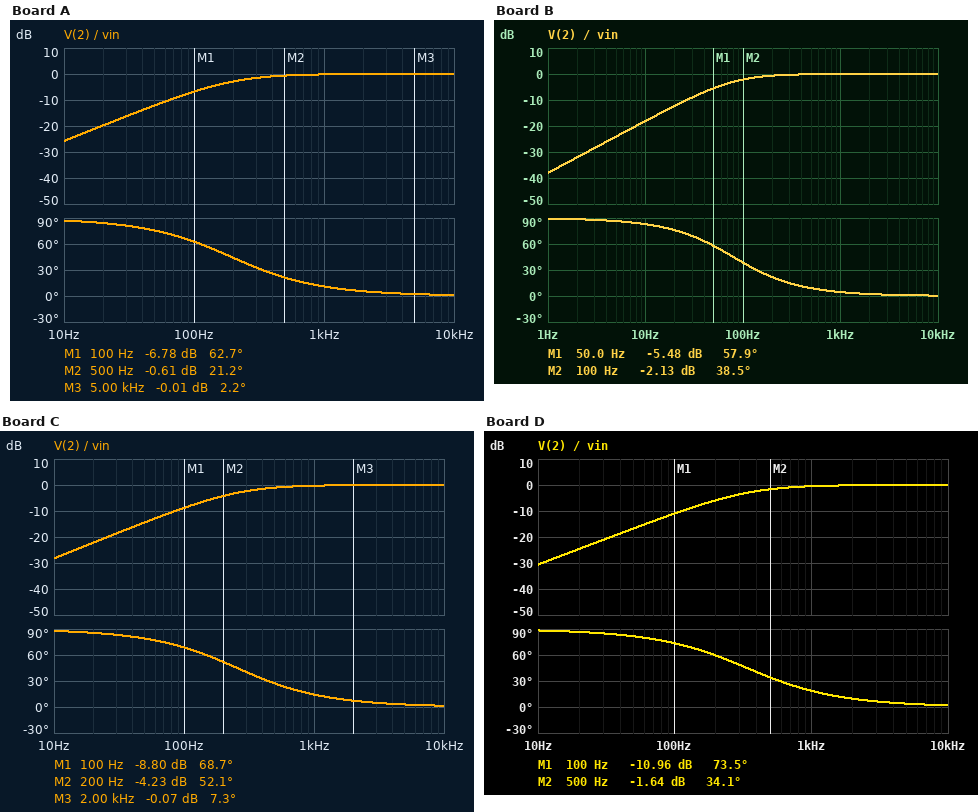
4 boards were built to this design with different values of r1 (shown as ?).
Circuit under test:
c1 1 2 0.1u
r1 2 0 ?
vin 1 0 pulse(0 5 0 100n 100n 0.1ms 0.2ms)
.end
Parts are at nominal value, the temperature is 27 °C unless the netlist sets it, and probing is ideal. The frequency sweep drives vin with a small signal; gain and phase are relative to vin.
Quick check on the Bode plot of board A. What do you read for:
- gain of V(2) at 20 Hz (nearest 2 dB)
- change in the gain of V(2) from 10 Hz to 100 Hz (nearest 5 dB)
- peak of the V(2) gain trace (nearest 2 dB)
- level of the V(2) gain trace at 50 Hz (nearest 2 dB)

-20 dB
20 dB
0 dB
-12 dB
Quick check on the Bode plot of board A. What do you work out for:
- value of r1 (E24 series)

8.2 kΩ
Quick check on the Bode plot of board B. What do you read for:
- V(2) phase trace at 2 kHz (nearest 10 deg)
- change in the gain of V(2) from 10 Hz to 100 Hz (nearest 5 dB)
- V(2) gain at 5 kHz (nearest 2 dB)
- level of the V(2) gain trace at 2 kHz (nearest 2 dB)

0 deg
15 dB
0 dB
0 dB
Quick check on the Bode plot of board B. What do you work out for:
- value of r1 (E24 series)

20 kΩ
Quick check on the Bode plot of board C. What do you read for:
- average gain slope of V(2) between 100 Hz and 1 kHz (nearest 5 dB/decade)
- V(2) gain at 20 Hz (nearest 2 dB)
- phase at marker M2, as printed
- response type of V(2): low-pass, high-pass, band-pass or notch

10 dB/decade
-22 dB
52.1 deg
high-pass
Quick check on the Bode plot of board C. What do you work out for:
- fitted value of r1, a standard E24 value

6.2 kΩ
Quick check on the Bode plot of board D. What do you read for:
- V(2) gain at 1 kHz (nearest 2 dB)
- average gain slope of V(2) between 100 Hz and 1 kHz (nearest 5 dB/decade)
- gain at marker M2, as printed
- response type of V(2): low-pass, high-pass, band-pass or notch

0 dB
10 dB/decade
-1.64 dB
high-pass
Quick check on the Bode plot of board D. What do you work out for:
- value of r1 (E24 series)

4.7 kΩ
